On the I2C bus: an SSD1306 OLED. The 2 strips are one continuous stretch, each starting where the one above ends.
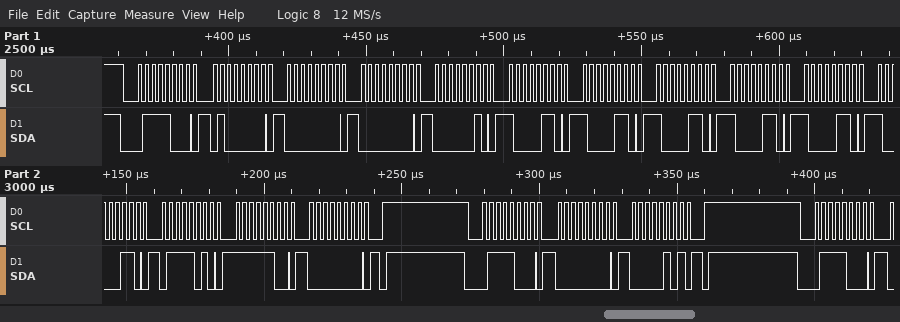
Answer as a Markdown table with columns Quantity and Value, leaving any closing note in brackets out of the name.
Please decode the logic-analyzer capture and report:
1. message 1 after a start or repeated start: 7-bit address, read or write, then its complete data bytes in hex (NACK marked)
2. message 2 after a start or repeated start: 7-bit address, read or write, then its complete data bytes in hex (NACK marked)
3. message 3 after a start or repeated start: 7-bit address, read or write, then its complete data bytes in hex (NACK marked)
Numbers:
| Quantity | Value |
|---|---|
| message 1 after a start or repeated start: 7-bit address, read or write, then its complete data bytes in hex | 0x3C write: 40 00 00 02 86 86 86 86 86 86 7A FC 00 |
| message 2 after a start or repeated start: 7-bit address, read or write, then its complete data bytes in hex | 0x3C write: 00 05 |
| message 3 after a start or repeated start: 7-bit address, read or write, then its complete data bytes in hex | 0x3C write |
